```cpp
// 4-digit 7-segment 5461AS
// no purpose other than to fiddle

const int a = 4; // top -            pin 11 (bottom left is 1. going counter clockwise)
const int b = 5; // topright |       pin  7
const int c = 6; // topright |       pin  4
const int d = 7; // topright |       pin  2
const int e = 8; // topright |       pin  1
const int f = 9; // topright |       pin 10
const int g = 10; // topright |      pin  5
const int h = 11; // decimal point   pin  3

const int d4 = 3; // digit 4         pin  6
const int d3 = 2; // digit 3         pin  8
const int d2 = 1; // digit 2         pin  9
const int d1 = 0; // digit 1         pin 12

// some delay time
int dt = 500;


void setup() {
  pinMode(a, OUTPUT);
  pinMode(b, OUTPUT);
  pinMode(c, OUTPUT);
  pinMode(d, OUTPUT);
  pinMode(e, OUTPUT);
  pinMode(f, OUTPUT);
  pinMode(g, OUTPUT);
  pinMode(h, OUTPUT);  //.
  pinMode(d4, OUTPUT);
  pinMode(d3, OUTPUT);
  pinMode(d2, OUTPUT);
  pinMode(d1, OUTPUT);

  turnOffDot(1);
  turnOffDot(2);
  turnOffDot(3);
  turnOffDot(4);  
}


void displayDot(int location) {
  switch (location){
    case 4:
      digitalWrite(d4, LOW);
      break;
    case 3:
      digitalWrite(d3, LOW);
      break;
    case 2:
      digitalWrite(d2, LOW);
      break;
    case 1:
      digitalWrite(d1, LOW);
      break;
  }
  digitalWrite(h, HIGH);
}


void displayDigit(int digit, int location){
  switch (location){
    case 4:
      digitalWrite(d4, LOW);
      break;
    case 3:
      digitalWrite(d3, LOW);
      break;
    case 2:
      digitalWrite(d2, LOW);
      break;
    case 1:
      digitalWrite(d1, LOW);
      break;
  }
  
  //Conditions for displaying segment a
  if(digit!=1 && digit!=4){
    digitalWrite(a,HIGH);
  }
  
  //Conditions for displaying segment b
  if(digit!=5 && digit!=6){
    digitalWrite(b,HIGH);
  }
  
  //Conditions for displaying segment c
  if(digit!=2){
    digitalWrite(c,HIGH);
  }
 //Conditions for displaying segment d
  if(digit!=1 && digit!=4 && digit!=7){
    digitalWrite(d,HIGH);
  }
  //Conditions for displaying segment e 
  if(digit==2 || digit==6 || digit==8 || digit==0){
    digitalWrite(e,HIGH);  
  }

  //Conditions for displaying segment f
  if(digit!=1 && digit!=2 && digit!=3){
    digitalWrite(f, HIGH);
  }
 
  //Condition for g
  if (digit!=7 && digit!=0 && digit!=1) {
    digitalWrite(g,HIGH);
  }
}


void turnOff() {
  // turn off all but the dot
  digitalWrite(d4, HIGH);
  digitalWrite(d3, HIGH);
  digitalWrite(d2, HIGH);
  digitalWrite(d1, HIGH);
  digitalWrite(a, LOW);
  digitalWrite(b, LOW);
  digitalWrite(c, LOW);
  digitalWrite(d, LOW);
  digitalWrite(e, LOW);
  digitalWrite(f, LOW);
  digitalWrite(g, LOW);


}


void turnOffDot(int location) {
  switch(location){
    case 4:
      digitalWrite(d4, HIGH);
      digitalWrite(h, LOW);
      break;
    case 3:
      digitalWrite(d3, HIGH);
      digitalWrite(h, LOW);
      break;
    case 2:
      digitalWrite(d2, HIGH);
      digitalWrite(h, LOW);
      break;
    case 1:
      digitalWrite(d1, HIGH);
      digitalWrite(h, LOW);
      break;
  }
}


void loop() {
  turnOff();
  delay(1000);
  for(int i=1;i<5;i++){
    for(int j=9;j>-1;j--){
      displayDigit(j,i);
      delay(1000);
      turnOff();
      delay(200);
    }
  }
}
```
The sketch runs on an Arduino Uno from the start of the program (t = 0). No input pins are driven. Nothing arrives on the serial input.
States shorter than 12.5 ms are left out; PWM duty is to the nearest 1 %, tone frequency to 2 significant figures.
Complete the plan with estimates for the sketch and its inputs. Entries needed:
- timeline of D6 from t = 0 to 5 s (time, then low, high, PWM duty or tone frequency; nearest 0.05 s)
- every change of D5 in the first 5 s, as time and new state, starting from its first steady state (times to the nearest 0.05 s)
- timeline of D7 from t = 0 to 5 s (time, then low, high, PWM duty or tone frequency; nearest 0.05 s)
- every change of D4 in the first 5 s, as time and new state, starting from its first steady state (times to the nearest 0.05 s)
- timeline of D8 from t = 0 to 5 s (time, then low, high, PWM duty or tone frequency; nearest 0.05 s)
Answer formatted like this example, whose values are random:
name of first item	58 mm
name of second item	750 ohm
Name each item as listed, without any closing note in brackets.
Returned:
timeline of D6 from t = 0 to 5 s	0 s low; 1 s high; 2 s low; 2.2 s high; 3.2 s low; 3.4 s high; 4.4 s low; 4.6 s high
every change of D5 in the first 5 s, as time and new state, starting from its first steady state	0 s low; 1 s high; 2 s low; 2.2 s high; 3.2 s low; 3.4 s high; 4.4 s low
timeline of D7 from t = 0 to 5 s	0 s low; 1 s high; 2 s low; 2.2 s high; 3.2 s low; 4.6 s high
every change of D4 in the first 5 s, as time and new state, starting from its first steady state	0 s low; 1 s high; 2 s low; 2.2 s high; 3.2 s low; 3.4 s high; 4.4 s low; 4.6 s high
timeline of D8 from t = 0 to 5 s	0 s low; 2.2 s high; 3.2 s low; 4.6 s high
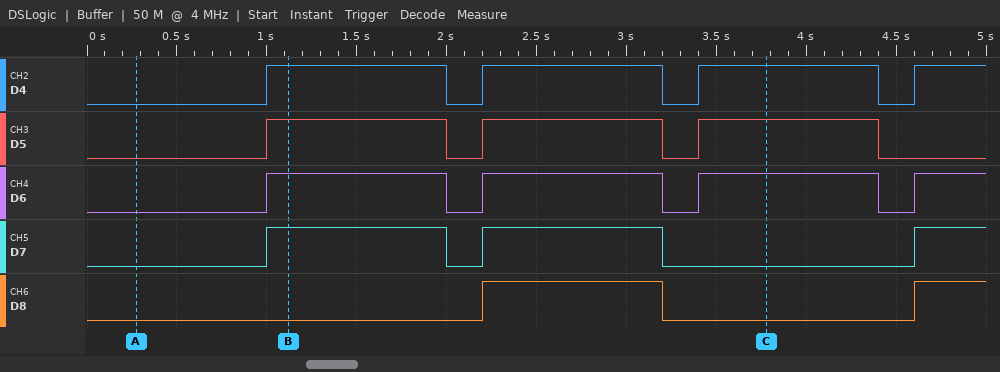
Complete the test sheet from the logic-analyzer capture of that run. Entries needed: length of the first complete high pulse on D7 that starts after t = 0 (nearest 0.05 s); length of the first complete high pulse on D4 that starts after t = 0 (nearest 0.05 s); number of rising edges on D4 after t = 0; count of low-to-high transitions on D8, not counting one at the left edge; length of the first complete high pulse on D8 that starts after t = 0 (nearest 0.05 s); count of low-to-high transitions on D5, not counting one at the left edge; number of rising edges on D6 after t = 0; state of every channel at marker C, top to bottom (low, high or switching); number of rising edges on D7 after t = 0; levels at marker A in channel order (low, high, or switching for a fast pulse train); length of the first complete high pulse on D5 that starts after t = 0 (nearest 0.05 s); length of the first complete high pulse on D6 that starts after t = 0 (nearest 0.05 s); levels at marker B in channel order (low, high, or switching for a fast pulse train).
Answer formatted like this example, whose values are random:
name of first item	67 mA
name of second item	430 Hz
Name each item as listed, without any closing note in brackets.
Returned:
length of the first complete high pulse on D7 that starts after t = 0	1.00 s
length of the first complete high pulse on D4 that starts after t = 0	1.00 s
number of rising edges on D4 after t = 0	4
count of low-to-high transitions on D8, not counting one at the left edge	2
length of the first complete high pulse on D8 that starts after t = 0	1.00 s
count of low-to-high transitions on D5, not counting one at the left edge	3
number of rising edges on D6 after t = 0	4
state of every channel at marker C, top to bottom	D4 high, D5 high, D6 high, D7 low, D8 low
number of rising edges on D7 after t = 0	3
levels at marker A in channel order	D4 low, D5 low, D6 low, D7 low, D8 low
length of the first complete high pulse on D5 that starts after t = 0	1.00 s
length of the first complete high pulse on D6 that starts after t = 0	1.00 s
levels at marker B in channel order	D4 high, D5 high, D6 high, D7 high, D8 low
